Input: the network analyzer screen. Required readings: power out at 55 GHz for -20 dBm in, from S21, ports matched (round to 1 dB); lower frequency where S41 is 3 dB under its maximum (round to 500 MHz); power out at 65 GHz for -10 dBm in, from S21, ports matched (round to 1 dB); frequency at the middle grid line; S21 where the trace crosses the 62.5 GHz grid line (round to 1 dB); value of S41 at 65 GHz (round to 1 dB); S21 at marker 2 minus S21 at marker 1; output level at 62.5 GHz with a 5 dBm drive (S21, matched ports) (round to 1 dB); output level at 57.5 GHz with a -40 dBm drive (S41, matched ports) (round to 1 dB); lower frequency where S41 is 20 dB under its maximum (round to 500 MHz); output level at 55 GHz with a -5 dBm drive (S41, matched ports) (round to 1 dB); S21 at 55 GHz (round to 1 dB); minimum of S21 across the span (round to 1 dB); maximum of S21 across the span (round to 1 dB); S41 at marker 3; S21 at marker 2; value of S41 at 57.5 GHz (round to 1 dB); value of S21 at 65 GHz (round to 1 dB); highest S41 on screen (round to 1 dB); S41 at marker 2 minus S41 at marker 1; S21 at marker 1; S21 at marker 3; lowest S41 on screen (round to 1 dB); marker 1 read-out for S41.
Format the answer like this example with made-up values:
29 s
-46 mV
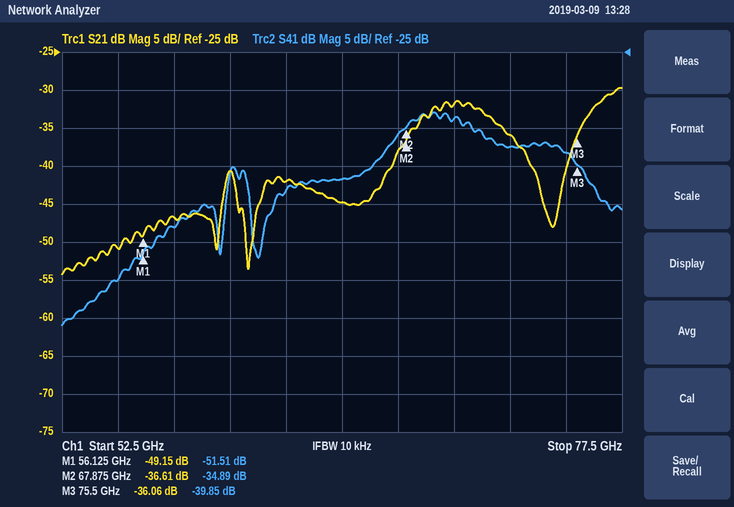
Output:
-71 dBm
67.5 GHz
-55 dBm
65 GHz
-42 dB
-42 dB
12.54 dB
-37 dBm
-88 dBm
55.5 GHz
-60 dBm
-51 dB
-54 dB
-30 dB
-39.85 dB
-36.61 dB
-48 dB
-45 dB
-33 dB
16.62 dB
-49.15 dB
-36.06 dB
-61 dB
-51.51 dB
